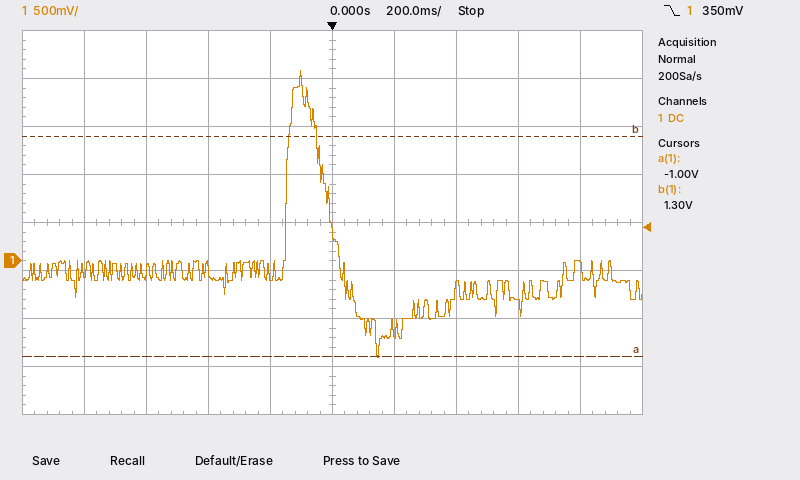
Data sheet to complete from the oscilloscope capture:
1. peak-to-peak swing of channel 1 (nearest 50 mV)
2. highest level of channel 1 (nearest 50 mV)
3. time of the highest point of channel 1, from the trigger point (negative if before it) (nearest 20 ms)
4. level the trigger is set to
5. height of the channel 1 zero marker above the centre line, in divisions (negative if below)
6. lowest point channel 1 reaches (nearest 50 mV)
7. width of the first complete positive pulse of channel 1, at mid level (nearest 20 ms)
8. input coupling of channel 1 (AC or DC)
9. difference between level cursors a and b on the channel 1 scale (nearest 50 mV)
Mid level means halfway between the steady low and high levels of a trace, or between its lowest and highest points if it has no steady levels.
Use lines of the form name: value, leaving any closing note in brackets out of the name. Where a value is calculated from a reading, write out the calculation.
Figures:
peak-to-peak swing of channel 1: 2.00 V − (-1.00 V) = 3.00 V
highest level of channel 1: 2.00 V
time of the highest point of channel 1, from the trigger point (negative if before it): -100 ms
level the trigger is set to: 350 mV
height of the channel 1 zero marker above the centre line, in divisions: -0.8 div
lowest point channel 1 reaches: -1.00 V
width of the first complete positive pulse of channel 1, at mid level: 140 ms
input coupling of channel 1: DC
difference between level cursors a and b on the channel 1 scale: 2.30 V
